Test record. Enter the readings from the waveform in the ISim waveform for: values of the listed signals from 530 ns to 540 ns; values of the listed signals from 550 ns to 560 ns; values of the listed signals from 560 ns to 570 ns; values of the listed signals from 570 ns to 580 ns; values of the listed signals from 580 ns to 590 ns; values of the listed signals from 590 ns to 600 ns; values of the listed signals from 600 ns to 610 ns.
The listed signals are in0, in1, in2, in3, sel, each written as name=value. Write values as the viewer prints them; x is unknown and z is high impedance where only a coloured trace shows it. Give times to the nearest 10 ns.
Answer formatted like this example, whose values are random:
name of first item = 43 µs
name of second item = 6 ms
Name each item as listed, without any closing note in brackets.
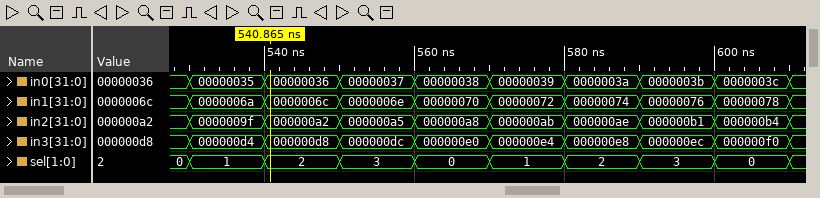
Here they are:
values of the listed signals from 530 ns to 540 ns = in0=00000035, in1=0000006a, in2=0000009f, in3=000000d4, sel=1
values of the listed signals from 550 ns to 560 ns = in0=00000037, in1=0000006e, in2=000000a5, in3=000000dc, sel=3
values of the listed signals from 560 ns to 570 ns = in0=00000038, in1=00000070, in2=000000a8, in3=000000e0, sel=0
values of the listed signals from 570 ns to 580 ns = in0=00000039, in1=00000072, in2=000000ab, in3=000000e4, sel=1
values of the listed signals from 580 ns to 590 ns = in0=0000003a, in1=00000074, in2=000000ae, in3=000000e8, sel=2
values of the listed signals from 590 ns to 600 ns = in0=0000003b, in1=00000076, in2=000000b1, in3=000000ec, sel=3
values of the listed signals from 600 ns to 610 ns = in0=0000003c, in1=00000078, in2=000000b4, in3=000000f0, sel=0
